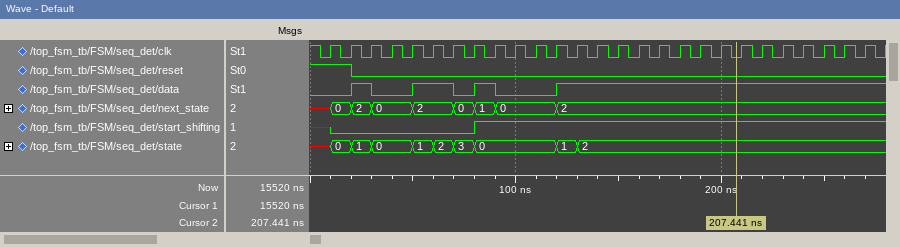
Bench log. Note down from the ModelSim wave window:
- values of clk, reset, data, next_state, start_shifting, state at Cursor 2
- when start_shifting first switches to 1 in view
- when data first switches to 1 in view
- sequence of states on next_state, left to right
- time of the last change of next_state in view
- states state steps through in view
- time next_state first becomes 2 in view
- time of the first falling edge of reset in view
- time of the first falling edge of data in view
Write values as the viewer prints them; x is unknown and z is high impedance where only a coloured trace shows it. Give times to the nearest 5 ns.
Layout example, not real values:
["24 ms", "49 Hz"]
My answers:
["clk=0, reset=0, data=1, next_state=2, start_shifting=1, state=2", "80 ns", "20 ns", "x, 0, 2, 0, 2, 0, 1, 0, 2", "120 ns", "x, 0, 1, 0, 1, 2, 3, 0, 1, 2", "20 ns", "20 ns", "30 ns"]
